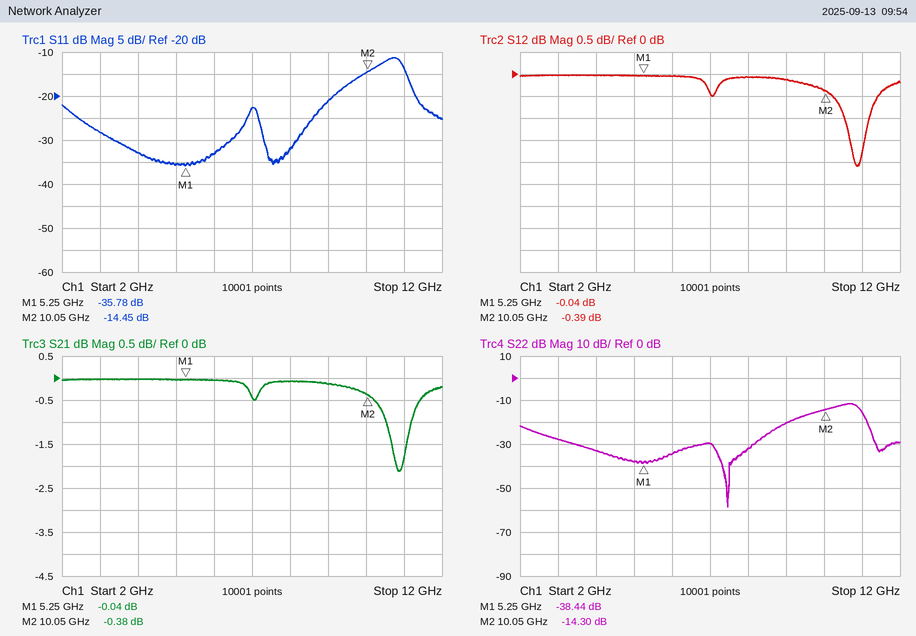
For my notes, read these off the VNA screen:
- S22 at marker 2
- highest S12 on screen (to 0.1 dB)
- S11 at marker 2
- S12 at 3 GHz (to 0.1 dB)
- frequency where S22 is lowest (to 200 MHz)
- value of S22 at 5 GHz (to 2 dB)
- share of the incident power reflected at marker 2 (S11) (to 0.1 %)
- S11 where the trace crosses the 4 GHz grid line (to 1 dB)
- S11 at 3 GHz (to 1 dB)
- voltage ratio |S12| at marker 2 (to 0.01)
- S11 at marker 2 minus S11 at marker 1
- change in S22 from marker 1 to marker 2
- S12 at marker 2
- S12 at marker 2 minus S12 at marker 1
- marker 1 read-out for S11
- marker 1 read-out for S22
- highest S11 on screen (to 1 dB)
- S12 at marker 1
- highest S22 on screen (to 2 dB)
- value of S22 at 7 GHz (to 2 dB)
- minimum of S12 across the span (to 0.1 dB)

-14.30 dB
0.0 dB
-14.45 dB
0.0 dB
7.4 GHz
-38 dB
3.6 %
-33 dB
-28 dB
0.96
21.33 dB
24.14 dB
-0.39 dB
-0.35 dB
-35.78 dB
-38.44 dB
-11 dB
-0.04 dB
-12 dB
-30 dB
-2.1 dB
